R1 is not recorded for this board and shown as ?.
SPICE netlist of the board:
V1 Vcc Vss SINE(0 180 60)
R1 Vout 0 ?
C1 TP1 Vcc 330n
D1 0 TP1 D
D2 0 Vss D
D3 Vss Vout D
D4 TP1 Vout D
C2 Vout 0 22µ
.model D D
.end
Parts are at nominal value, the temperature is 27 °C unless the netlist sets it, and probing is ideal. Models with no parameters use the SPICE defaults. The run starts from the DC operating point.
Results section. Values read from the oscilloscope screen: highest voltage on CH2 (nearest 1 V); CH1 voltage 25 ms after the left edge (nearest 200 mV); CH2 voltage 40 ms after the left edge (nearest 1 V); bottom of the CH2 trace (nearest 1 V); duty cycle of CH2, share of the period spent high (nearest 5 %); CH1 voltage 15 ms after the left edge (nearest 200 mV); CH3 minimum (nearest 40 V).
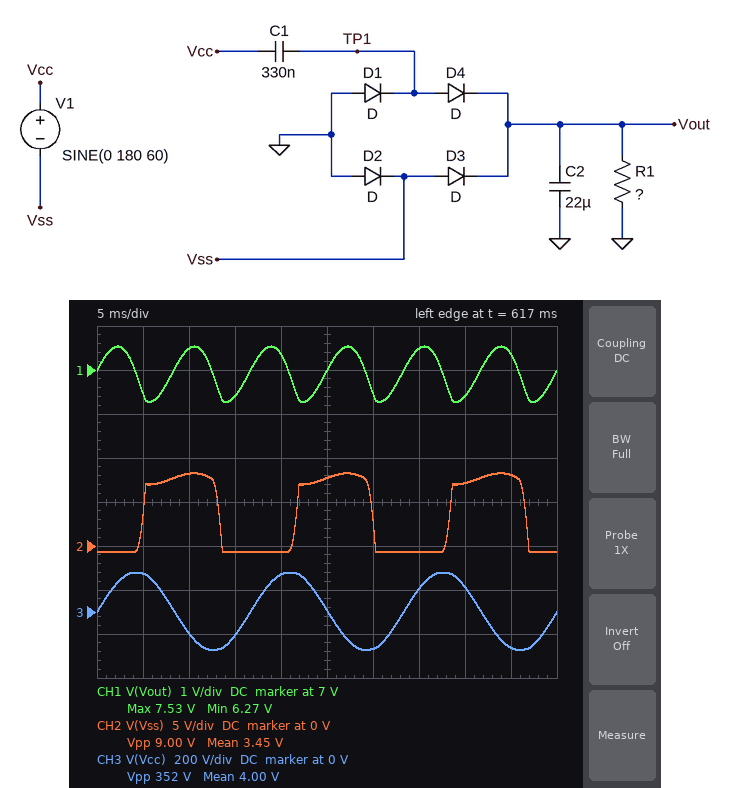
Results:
8 V
7.0 V
7 V
-1 V
50 %
6.4 V
-160 V
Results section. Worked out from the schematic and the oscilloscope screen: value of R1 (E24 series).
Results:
510 Ω
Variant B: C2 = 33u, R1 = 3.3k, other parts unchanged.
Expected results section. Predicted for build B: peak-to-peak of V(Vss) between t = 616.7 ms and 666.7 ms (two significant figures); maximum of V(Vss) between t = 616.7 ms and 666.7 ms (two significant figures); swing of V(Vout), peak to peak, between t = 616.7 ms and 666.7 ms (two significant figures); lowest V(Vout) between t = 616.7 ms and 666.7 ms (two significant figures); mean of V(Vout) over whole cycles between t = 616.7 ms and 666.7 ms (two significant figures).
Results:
39 V
38 V
1.1 V
36 V
37 V
